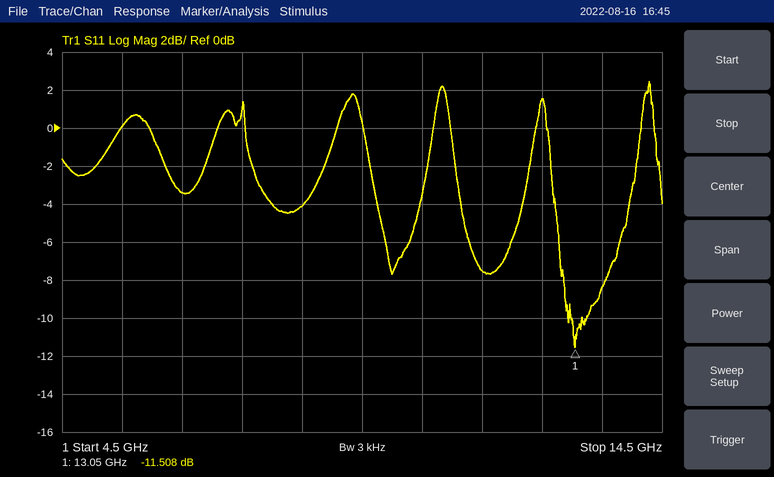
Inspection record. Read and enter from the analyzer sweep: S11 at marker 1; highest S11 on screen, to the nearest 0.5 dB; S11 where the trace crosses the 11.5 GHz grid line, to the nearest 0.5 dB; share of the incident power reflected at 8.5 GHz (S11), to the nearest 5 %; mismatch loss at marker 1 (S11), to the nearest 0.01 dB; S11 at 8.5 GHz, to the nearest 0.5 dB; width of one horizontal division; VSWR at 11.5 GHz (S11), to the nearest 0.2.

-11.508 dB
2.5 dB
-7.5 dB
40 %
0.32 dB
-4.0 dB
1 GHz
2.4
